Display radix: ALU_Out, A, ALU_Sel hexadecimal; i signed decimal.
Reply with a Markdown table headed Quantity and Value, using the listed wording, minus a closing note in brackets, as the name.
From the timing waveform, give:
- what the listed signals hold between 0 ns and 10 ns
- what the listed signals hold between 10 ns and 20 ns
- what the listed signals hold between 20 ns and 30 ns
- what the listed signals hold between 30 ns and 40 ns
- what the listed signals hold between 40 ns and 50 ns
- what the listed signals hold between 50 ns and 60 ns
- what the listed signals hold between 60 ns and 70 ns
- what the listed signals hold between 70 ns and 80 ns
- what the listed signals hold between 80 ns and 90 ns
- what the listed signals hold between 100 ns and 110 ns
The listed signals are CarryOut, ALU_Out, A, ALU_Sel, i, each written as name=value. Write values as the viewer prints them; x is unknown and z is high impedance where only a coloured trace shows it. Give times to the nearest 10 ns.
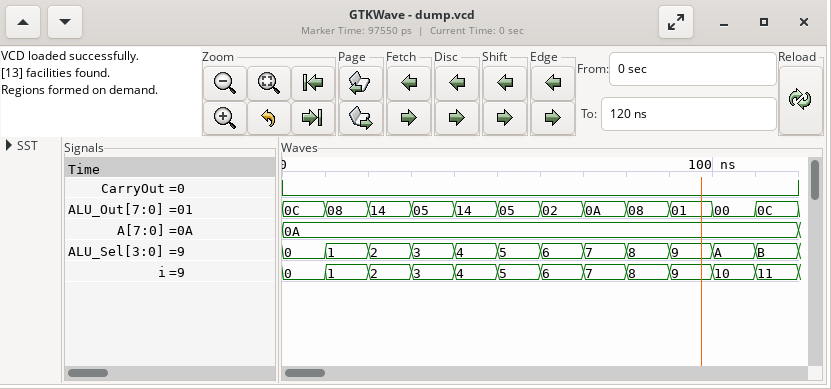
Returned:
| Quantity | Value |
|---|---|
| what the listed signals hold between 0 ns and 10 ns | CarryOut=0, ALU_Out=0C, A=0A, ALU_Sel=0, i=0 |
| what the listed signals hold between 10 ns and 20 ns | CarryOut=0, ALU_Out=08, A=0A, ALU_Sel=1, i=1 |
| what the listed signals hold between 20 ns and 30 ns | CarryOut=0, ALU_Out=14, A=0A, ALU_Sel=2, i=2 |
| what the listed signals hold between 30 ns and 40 ns | CarryOut=0, ALU_Out=05, A=0A, ALU_Sel=3, i=3 |
| what the listed signals hold between 40 ns and 50 ns | CarryOut=0, ALU_Out=14, A=0A, ALU_Sel=4, i=4 |
| what the listed signals hold between 50 ns and 60 ns | CarryOut=0, ALU_Out=05, A=0A, ALU_Sel=5, i=5 |
| what the listed signals hold between 60 ns and 70 ns | CarryOut=0, ALU_Out=02, A=0A, ALU_Sel=6, i=6 |
| what the listed signals hold between 70 ns and 80 ns | CarryOut=0, ALU_Out=0A, A=0A, ALU_Sel=7, i=7 |
| what the listed signals hold between 80 ns and 90 ns | CarryOut=0, ALU_Out=08, A=0A, ALU_Sel=8, i=8 |
| what the listed signals hold between 100 ns and 110 ns | CarryOut=0, ALU_Out=00, A=0A, ALU_Sel=A, i=10 |
